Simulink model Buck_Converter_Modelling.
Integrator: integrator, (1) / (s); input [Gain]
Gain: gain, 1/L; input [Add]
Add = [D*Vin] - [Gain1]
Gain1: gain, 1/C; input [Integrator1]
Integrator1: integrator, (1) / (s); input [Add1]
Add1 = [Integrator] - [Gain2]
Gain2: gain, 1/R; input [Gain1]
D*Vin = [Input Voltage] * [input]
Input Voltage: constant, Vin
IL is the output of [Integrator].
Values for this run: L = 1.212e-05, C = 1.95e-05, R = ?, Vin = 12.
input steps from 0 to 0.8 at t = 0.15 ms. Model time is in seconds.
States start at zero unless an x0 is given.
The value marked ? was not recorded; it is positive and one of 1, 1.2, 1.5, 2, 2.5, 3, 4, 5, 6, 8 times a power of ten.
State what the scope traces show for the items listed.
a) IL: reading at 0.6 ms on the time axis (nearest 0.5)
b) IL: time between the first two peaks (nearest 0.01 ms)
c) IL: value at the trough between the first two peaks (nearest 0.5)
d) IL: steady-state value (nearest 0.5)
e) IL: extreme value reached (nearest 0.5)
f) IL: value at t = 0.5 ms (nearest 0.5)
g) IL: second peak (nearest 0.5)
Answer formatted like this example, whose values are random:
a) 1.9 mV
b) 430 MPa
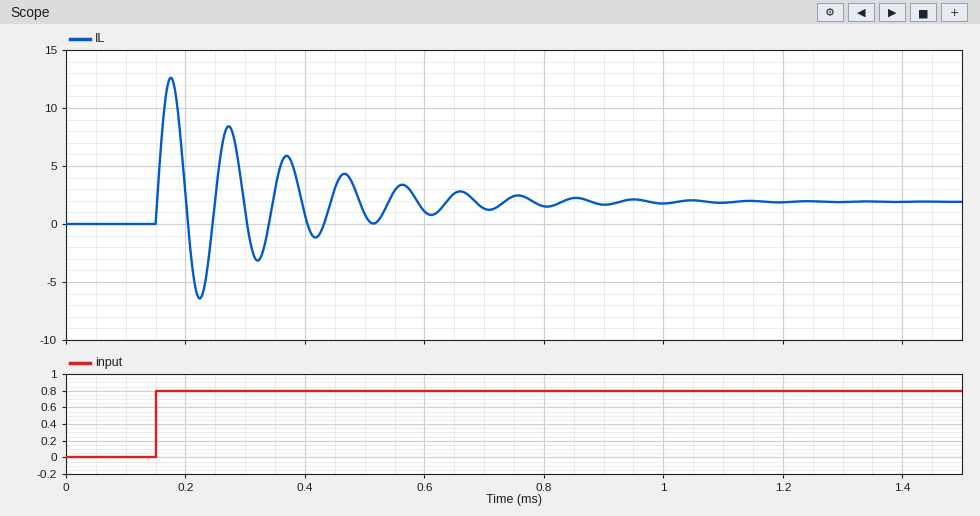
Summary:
a) 1.0
b) 0.10 ms
c) -6.5
d) 2.0
e) 12.5
f) 1.0
g) 8.5
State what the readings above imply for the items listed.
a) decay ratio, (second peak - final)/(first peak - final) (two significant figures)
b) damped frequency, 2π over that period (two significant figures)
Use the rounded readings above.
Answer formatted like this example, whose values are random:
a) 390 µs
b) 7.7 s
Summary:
a) 0.62
b) 63 rad/ms
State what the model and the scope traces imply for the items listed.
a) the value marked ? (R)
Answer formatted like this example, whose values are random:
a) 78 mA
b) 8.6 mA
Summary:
a) 5
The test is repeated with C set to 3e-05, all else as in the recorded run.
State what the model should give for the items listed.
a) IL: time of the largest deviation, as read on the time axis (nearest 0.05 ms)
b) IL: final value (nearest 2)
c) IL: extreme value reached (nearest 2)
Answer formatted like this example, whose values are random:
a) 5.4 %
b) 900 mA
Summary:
a) 0.20 ms
b) 2
c) 16
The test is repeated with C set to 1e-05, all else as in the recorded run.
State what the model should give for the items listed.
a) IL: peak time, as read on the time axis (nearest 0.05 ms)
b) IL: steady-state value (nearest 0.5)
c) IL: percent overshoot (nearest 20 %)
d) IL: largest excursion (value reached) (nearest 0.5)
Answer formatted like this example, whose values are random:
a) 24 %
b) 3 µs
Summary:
a) 0.15 ms
b) 2.0
c) 380 %
d) 9.0
